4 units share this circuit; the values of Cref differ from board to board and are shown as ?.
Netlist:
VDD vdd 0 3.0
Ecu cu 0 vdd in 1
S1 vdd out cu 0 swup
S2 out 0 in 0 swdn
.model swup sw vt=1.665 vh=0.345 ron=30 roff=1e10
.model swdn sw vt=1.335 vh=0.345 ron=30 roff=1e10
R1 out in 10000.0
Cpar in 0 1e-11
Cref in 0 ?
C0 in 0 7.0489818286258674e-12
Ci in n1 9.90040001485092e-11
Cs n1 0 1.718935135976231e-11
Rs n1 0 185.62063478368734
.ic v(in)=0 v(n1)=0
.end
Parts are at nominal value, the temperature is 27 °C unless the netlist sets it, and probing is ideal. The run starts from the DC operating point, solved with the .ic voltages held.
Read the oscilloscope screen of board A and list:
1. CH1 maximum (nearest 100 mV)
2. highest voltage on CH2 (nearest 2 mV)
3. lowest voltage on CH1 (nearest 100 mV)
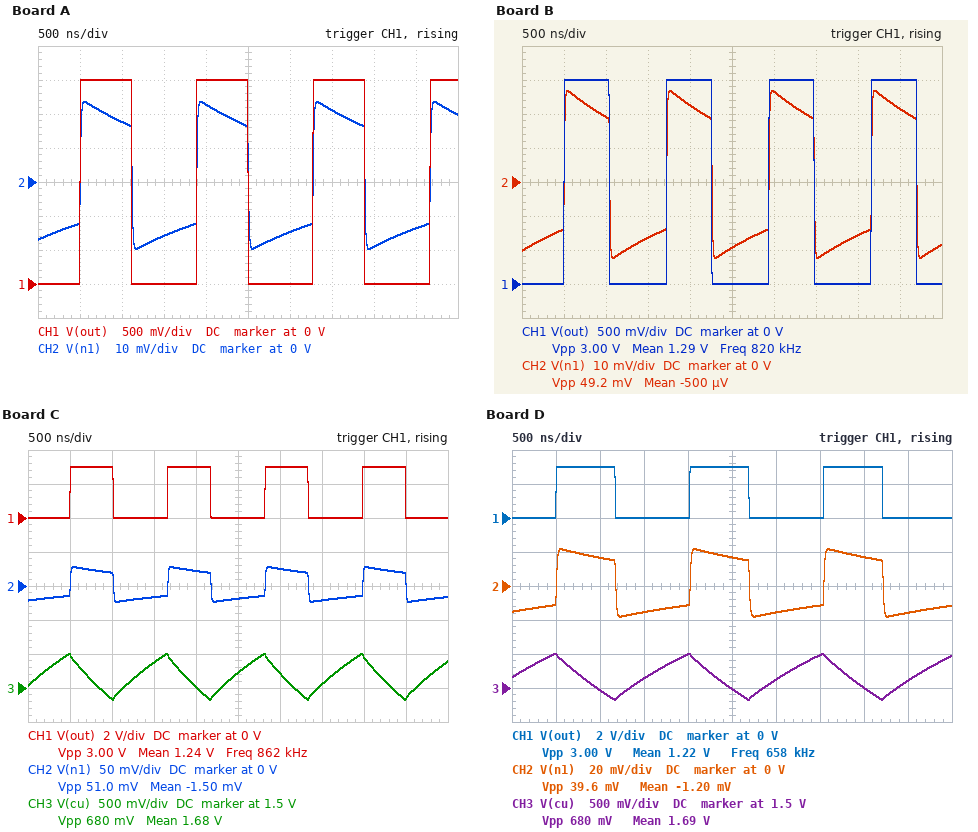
3.0 V
24 mV
0 V
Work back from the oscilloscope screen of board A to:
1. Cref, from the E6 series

33 pF
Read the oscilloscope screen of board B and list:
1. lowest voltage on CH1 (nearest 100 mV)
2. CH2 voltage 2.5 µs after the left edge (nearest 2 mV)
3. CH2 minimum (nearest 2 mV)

0 V
-20 mV
-22 mV
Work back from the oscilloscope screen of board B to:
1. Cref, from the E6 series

15 pF
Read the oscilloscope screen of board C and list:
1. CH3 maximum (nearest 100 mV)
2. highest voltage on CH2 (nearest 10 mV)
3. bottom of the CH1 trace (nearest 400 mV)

2.0 V
30 mV
0 V
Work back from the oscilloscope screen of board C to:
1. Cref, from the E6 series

10 pF
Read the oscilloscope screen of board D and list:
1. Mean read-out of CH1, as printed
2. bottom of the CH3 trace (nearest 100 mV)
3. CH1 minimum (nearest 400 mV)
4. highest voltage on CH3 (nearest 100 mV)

1.22 V
1.3 V
0 V
2.0 V
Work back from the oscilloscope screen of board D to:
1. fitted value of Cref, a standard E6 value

47 pF
